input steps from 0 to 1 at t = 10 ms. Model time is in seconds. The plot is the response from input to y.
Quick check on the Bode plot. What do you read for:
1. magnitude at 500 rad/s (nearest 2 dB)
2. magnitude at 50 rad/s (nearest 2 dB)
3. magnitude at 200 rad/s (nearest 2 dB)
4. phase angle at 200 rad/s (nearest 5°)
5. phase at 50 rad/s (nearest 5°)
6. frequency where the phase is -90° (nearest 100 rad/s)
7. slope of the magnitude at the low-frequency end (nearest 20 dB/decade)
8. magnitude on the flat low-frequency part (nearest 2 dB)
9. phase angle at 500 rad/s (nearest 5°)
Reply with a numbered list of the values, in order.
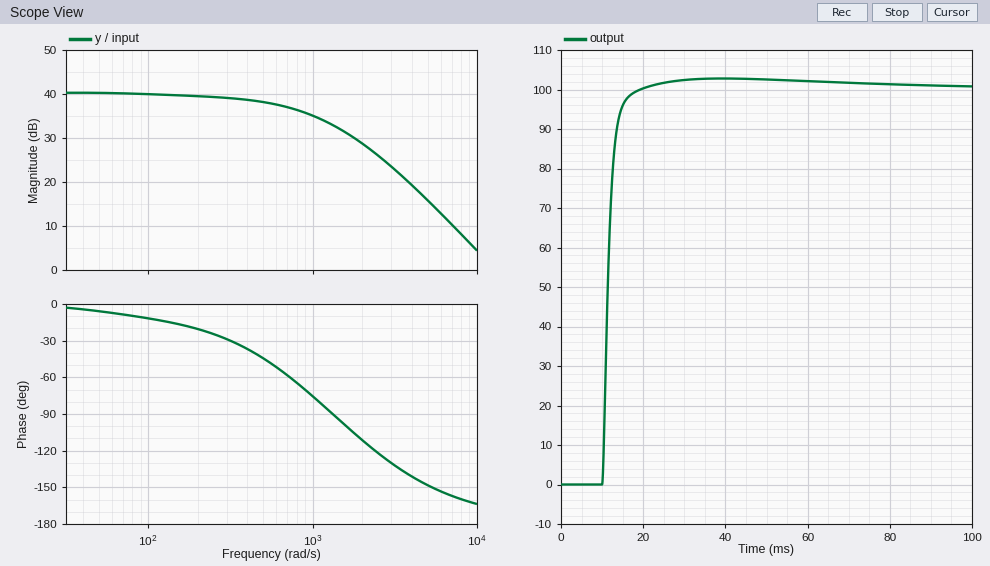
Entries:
1. 38 dB
2. 40 dB
3. 40 dB
4. -20°
5. -5°
6. 1300 rad/s
7. 0 dB/decade
8. 40 dB
9. -45°
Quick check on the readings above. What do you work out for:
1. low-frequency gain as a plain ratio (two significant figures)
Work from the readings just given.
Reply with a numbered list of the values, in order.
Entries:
1. 100
